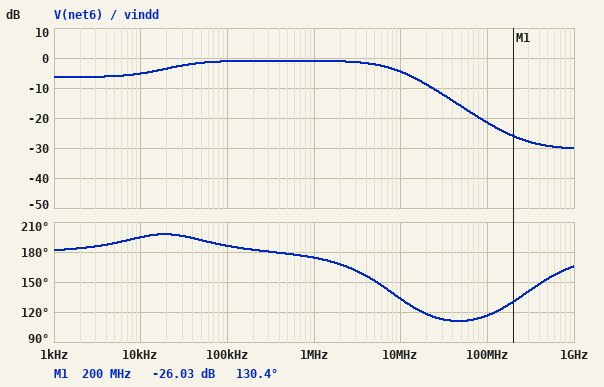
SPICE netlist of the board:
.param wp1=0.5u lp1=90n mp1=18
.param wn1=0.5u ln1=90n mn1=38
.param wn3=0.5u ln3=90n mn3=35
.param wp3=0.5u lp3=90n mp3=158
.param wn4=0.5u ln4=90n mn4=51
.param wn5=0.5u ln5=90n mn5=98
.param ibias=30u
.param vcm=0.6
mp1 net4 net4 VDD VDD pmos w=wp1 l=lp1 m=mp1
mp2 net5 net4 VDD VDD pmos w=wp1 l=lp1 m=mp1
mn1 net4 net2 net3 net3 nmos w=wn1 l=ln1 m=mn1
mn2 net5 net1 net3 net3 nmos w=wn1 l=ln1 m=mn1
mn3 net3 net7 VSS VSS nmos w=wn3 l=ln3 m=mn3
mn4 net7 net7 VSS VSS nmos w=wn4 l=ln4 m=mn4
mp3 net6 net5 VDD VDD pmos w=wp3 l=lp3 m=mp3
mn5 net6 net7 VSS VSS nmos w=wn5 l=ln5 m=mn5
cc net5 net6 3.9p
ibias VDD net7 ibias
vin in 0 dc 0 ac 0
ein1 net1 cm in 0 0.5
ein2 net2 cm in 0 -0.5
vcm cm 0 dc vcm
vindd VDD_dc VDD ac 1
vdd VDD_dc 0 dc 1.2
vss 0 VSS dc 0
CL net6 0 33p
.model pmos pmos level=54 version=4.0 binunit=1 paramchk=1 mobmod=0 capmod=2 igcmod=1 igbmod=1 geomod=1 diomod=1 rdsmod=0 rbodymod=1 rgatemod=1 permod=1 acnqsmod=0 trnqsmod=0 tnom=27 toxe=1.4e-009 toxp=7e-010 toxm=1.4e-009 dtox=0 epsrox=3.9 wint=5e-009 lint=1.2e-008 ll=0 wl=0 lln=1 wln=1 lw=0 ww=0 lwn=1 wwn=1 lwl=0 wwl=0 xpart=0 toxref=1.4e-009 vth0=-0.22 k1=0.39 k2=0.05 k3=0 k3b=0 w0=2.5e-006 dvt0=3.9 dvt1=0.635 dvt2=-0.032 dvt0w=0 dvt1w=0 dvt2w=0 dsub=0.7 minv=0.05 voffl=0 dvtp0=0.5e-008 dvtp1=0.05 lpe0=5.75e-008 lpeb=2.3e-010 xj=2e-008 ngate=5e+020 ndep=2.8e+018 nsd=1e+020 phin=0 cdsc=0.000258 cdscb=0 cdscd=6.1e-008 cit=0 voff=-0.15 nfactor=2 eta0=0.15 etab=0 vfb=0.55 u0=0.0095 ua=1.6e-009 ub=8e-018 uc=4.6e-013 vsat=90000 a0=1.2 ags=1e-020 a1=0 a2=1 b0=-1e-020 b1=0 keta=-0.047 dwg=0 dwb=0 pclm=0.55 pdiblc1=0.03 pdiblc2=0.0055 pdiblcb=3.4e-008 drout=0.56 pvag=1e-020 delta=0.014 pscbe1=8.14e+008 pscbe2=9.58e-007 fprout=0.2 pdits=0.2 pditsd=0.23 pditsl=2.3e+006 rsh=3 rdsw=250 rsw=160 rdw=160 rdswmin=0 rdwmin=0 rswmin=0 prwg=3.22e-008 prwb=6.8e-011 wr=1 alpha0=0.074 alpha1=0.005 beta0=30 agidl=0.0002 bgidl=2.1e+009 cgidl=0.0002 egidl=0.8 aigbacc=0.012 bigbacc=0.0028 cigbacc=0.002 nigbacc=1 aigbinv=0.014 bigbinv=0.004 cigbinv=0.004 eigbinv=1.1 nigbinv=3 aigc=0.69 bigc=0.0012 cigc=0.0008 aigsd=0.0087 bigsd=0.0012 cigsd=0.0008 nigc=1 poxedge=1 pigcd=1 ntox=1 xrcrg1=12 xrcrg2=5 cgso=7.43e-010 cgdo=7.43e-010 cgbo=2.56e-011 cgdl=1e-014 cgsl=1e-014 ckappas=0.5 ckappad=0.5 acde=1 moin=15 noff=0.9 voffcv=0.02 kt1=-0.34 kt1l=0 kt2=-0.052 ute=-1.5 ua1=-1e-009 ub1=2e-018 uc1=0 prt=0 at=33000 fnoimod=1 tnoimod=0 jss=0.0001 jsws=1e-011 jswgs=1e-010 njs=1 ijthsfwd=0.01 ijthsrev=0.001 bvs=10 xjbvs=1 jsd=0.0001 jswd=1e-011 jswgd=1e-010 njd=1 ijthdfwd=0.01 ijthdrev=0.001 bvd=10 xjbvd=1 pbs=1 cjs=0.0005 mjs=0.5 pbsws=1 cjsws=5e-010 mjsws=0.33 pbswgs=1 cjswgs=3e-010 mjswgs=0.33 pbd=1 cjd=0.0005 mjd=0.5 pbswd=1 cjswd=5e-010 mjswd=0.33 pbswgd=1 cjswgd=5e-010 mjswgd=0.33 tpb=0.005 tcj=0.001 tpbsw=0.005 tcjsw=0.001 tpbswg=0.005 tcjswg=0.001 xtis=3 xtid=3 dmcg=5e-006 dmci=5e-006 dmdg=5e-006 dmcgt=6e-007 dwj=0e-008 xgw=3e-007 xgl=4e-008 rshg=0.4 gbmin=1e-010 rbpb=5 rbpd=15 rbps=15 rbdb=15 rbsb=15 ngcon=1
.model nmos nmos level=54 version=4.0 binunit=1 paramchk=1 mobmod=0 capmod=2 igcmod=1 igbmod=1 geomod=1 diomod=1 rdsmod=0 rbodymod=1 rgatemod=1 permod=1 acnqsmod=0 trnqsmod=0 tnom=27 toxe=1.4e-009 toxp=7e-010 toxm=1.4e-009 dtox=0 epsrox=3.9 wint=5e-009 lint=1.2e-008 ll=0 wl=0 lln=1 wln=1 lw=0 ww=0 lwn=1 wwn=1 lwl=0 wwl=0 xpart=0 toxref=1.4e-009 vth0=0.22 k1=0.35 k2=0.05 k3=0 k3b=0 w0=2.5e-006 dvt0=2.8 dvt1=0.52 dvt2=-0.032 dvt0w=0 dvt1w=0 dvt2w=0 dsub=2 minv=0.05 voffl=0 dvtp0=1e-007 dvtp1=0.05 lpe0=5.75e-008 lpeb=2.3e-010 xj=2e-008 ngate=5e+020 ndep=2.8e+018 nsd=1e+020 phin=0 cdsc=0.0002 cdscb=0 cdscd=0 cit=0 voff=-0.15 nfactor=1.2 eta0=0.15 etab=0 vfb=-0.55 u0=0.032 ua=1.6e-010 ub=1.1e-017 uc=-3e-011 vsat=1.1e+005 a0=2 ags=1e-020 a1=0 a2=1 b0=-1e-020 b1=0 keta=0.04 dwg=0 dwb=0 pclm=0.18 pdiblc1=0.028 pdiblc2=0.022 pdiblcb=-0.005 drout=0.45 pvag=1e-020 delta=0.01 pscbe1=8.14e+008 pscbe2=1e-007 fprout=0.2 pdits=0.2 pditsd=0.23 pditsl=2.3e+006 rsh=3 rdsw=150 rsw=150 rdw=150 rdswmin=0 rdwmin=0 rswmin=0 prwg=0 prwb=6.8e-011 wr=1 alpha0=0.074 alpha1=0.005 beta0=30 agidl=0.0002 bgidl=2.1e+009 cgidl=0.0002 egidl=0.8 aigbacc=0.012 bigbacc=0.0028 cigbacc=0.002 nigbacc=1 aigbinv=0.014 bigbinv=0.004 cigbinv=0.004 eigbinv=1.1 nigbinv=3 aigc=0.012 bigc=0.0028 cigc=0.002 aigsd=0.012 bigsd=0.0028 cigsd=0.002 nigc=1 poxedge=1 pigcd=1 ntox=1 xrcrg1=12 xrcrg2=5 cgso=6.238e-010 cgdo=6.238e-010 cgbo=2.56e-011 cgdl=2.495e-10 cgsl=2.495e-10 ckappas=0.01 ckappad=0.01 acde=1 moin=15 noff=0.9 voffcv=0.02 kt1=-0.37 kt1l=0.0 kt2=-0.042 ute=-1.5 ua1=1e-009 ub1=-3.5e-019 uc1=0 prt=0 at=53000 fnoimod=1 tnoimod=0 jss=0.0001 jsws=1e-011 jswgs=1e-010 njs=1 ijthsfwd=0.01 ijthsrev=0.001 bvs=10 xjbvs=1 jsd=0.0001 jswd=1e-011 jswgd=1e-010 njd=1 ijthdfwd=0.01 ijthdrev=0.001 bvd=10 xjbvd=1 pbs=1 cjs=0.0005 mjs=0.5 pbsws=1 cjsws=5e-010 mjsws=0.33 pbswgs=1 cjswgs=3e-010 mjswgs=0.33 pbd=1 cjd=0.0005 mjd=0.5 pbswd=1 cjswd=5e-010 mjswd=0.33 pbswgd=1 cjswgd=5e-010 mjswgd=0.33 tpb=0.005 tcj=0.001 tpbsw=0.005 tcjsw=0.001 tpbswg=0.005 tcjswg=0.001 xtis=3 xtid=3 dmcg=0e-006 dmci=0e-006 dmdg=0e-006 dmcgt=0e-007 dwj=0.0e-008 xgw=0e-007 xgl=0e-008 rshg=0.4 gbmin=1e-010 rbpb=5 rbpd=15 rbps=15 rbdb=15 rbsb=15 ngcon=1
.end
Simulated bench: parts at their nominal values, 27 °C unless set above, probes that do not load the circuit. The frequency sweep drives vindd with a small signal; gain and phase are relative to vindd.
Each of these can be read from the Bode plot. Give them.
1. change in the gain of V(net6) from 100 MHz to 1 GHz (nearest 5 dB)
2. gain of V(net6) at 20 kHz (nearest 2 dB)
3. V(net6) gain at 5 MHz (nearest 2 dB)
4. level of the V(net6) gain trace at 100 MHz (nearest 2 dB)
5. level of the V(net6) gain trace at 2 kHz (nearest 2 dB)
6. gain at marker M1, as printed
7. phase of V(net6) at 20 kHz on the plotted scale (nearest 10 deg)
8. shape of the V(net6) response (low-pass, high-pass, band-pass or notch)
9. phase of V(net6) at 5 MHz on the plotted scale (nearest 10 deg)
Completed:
-10 dB
-4 dB
-2 dB
-22 dB
-6 dB
-26.03 dB
200 deg
low-pass
150 deg
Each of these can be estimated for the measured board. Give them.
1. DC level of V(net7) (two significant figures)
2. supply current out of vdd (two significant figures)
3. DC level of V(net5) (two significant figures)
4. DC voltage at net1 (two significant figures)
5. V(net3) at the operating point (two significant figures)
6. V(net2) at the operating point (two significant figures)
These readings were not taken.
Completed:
300 mV
140 µA
870 mV
600 mV
340 mV
600 mV
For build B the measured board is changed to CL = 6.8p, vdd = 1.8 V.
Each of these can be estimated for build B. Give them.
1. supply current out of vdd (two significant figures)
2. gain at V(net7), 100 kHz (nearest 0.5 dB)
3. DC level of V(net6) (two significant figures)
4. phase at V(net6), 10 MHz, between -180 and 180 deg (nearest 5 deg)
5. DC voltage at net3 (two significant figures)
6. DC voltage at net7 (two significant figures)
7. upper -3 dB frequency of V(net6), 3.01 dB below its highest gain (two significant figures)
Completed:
210 µA
-26.0 dB
1.3 V
170 deg
350 mV
310 mV
58 MHz
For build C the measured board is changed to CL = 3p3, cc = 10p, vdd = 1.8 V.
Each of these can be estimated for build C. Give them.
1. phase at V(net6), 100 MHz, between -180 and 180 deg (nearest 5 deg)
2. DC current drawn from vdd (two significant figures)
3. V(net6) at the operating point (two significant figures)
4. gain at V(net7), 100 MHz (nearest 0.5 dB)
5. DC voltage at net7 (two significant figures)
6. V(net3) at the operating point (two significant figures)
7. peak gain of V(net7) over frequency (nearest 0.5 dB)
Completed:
150 deg
210 µA
1.3 V
-27.5 dB
310 mV
350 mV
-25.5 dB
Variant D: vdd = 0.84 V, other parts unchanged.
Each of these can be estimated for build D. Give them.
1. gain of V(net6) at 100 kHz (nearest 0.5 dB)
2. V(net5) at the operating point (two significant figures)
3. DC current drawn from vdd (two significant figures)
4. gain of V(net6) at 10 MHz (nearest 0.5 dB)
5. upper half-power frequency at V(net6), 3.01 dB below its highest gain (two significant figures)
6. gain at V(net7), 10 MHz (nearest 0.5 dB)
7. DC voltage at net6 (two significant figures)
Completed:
-1.5 dB
510 mV
130 µA
-5.0 dB
7.8 MHz
-49.5 dB
730 mV
